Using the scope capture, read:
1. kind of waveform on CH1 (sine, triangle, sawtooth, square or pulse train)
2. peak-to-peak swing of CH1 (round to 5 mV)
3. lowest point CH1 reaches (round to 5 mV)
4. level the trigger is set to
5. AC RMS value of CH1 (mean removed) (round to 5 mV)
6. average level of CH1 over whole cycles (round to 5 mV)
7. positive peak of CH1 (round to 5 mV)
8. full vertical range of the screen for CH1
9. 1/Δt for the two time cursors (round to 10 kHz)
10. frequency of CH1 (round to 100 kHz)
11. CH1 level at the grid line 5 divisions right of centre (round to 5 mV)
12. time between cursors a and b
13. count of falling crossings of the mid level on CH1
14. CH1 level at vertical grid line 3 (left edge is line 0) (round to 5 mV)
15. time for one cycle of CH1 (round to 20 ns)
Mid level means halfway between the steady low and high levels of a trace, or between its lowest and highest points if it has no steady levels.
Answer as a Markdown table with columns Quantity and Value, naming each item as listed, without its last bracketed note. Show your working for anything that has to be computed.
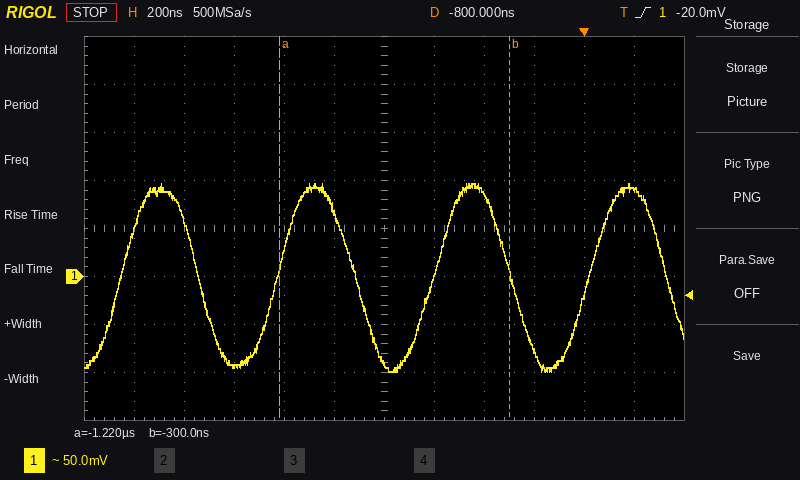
| Quantity | Value |
|---|---|
| kind of waveform on CH1 | sine |
| peak-to-peak swing of CH1 | 95 mV − (-100 mV) = 195 mV |
| lowest point CH1 reaches | -100 mV |
| level the trigger is set to | -20.0 mV |
| AC RMS value of CH1 (mean removed) | 195 mV / (2√2) ≈ 68.9 mV, so 70 mV to the nearest 5 mV |
| average level of CH1 over whole cycles | (95 mV + (-100 mV)) / 2 ≈ 0 mV |
| positive peak of CH1 | 95 mV |
| full vertical range of the screen for CH1 | 400 mV |
| 1/Δt for the two time cursors | 1 / 920 ns ≈ 1.09 MHz |
| frequency of CH1 | 1 / 620 ns ≈ 1.6 MHz |
| CH1 level at the grid line 5 divisions right of centre | 90 mV |
| time between cursors a and b | -300 ns − (-1.22 µs) = 920 ns |
| count of falling crossings of the mid level on CH1 | 4 |
| CH1 level at vertical grid line 3 (left edge is line 0) | -95 mV |
| time for one cycle of CH1 | 620 ns |
